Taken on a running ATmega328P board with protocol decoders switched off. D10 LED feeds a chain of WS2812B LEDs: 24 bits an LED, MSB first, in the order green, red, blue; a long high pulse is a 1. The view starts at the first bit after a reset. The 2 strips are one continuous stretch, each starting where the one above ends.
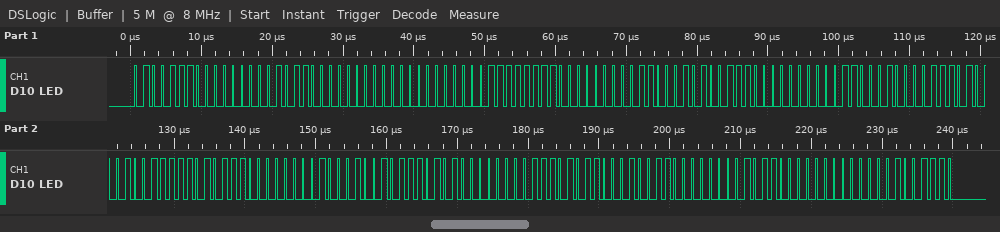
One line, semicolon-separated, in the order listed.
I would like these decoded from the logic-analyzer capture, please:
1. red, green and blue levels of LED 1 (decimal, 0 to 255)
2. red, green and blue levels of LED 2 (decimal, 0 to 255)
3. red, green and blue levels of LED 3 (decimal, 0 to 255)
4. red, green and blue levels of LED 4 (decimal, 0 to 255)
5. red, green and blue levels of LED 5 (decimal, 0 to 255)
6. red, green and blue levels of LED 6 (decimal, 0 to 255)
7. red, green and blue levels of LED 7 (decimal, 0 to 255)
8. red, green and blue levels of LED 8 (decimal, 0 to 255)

0, 78, 176; 0, 0, 255; 98, 0, 156; 196, 0, 58; 215, 39, 0; 117, 137, 0; 19, 235, 0; 0, 176, 78
